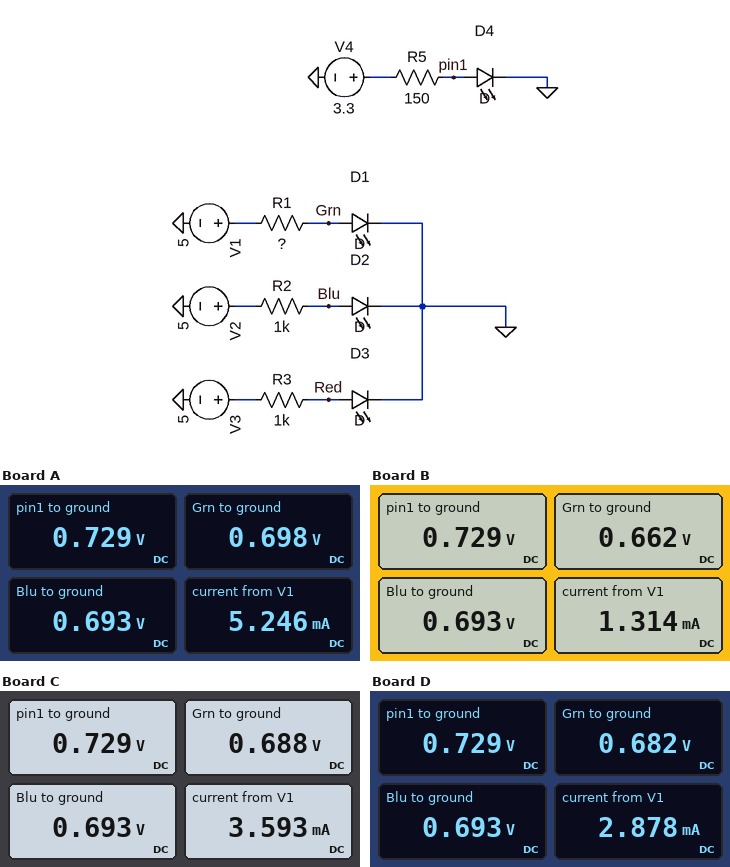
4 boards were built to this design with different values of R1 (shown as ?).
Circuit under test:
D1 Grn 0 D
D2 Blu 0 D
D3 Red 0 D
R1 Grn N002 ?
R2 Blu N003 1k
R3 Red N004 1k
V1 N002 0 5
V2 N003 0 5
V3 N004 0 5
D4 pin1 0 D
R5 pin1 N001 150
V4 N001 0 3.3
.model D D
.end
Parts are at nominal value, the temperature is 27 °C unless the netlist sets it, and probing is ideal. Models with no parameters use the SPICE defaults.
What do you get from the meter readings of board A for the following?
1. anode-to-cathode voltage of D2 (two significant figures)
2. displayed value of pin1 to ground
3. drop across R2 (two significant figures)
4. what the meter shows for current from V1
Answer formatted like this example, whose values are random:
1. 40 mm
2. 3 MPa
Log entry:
1. 690 mV
2. 0.729 V
3. 4.3 V
4. 5.246 mA
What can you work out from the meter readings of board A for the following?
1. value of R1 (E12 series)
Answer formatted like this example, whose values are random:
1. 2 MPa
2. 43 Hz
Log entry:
1. 820 Ω
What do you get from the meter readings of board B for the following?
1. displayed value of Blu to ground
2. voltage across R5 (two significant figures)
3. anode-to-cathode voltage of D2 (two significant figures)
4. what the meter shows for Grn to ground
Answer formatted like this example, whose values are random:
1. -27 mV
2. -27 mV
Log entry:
1. 0.693 V
2. 2.6 V
3. 690 mV
4. 0.662 V
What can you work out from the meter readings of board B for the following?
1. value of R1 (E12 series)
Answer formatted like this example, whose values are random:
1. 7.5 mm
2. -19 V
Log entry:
1. 3.3 kΩ
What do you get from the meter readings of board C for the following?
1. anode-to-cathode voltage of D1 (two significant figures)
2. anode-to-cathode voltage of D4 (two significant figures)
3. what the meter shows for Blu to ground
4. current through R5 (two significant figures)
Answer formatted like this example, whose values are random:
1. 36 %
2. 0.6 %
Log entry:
1. 690 mV
2. 730 mV
3. 0.693 V
4. 17 mA
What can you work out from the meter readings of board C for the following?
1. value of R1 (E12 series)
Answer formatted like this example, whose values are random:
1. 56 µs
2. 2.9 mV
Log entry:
1. 1.2 kΩ
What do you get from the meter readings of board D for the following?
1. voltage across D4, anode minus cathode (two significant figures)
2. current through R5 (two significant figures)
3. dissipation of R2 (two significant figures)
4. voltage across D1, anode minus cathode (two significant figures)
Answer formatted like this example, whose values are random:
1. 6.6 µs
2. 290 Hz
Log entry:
1. 730 mV
2. 17 mA
3. 19 mW
4. 680 mV
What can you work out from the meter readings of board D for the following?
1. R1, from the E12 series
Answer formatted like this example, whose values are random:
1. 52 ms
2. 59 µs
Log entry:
1. 1.5 kΩ
